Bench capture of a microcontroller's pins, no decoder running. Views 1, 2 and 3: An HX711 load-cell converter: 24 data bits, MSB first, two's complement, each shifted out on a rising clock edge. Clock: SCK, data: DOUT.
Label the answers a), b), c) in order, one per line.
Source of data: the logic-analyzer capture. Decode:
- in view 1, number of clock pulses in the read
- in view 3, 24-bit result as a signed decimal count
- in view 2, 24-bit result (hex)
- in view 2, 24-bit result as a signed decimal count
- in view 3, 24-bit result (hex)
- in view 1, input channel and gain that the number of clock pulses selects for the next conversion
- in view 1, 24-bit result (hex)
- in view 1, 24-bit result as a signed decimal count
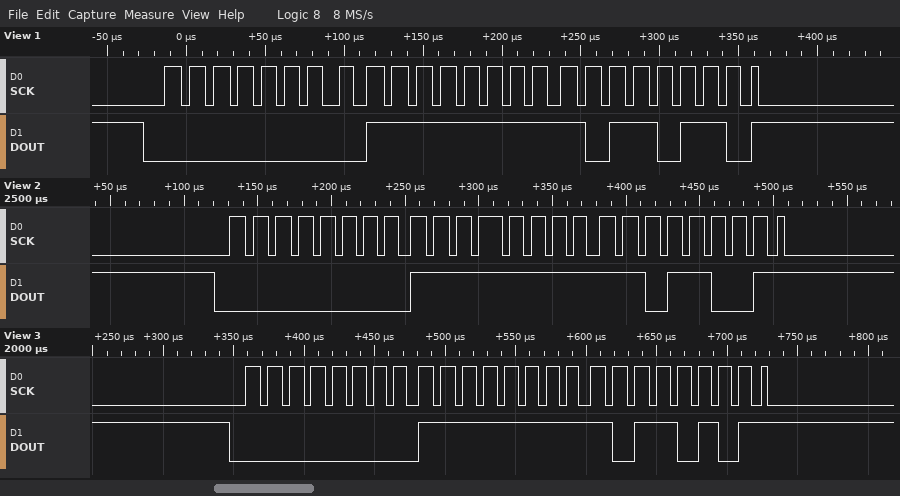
a) 25
b) 65461
c) 0x00FFD9
d) 65497
e) 0x00FFB5
f) channel A, gain 128
g) 0x00FFB6
h) 65462
